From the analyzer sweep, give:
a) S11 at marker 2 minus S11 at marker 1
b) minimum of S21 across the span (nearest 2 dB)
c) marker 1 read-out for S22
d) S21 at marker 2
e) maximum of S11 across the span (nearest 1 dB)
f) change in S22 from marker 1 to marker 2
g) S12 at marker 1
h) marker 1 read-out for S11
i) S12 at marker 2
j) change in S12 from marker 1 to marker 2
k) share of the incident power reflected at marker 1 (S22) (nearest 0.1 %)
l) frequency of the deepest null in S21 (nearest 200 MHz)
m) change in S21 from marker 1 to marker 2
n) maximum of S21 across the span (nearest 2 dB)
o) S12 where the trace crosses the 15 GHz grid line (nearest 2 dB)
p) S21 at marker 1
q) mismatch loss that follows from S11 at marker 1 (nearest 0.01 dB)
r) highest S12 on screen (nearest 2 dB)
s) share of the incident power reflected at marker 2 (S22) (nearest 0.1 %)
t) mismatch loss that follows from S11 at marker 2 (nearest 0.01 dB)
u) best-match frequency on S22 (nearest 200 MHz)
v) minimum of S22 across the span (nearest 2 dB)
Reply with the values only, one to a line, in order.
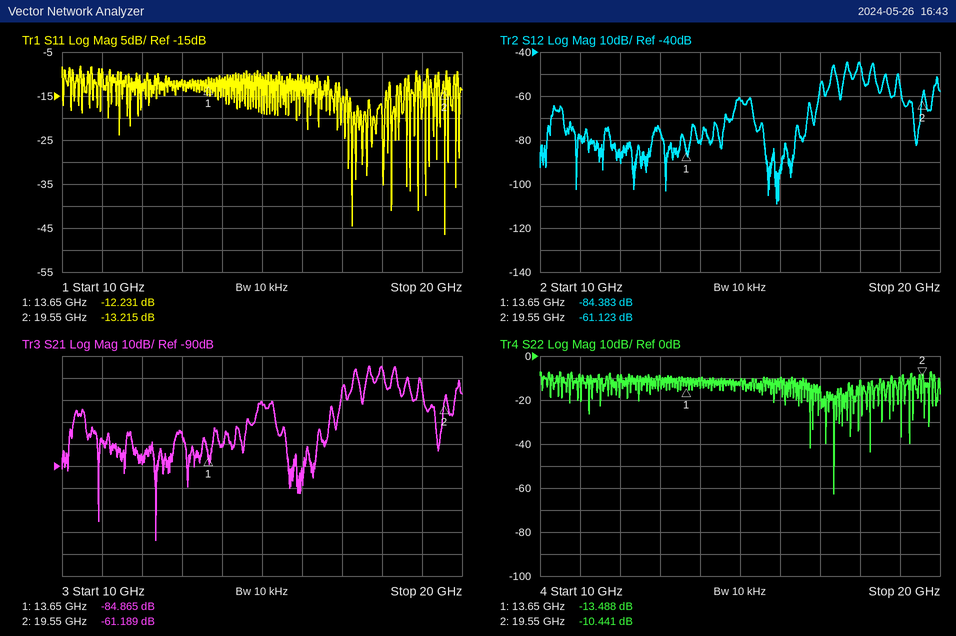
-0.984 dB
-124 dB
-13.488 dB
-61.189 dB
-8 dB
3.047 dB
-84.383 dB
-12.231 dB
-61.123 dB
23.260 dB
4.5 %
12.4 GHz
23.676 dB
-44 dB
-62 dB
-84.865 dB
0.27 dB
-44 dB
9.0 %
0.21 dB
17.4 GHz
-62 dB
